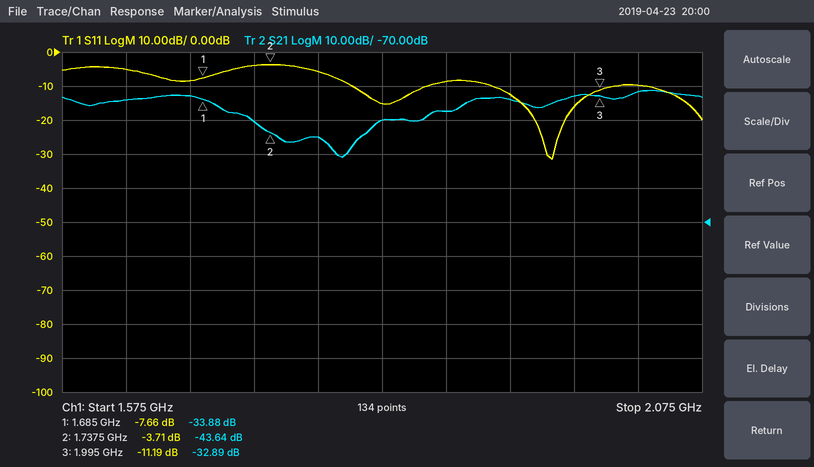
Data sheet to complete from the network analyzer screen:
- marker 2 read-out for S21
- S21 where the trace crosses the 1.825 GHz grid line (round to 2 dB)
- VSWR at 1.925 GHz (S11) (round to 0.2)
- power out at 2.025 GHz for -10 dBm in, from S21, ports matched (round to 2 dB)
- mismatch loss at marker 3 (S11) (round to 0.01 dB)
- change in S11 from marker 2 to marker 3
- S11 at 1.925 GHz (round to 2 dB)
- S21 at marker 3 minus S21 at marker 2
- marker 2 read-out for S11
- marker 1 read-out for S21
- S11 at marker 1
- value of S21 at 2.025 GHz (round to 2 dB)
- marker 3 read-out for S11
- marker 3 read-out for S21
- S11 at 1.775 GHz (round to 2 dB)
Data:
-43.64 dB
-40 dB
1.6
-42 dBm
0.34 dB
-7.48 dB
-12 dB
10.75 dB
-3.71 dB
-33.88 dB
-7.66 dB
-32 dB
-11.19 dB
-32.89 dB
-6 dB
